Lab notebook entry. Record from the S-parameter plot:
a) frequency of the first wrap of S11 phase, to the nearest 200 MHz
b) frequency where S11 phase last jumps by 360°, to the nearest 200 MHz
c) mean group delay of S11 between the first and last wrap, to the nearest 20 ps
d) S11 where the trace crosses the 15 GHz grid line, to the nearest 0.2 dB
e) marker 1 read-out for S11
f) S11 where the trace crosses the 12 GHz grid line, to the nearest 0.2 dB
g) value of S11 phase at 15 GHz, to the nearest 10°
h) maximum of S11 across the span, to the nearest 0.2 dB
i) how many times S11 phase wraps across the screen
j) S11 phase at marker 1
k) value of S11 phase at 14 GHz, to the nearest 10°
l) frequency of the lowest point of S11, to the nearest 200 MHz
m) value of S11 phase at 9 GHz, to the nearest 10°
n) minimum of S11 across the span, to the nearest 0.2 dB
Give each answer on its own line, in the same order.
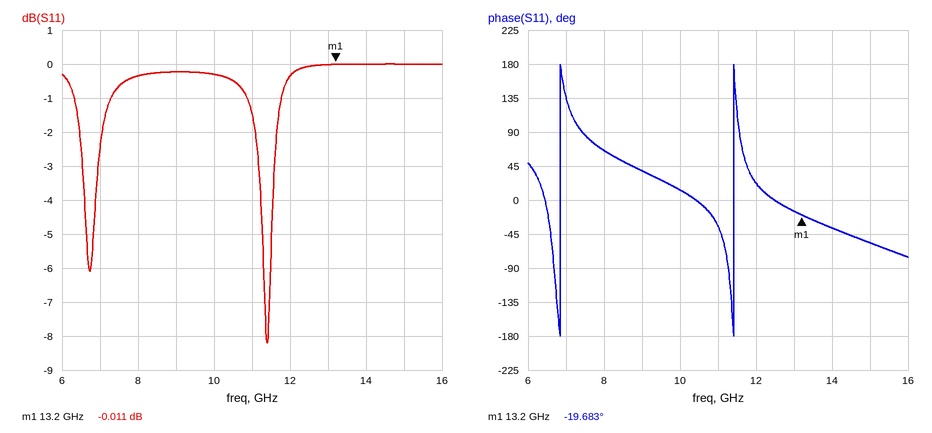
6.8 GHz
11.4 GHz
220 ps
0.0 dB
-0.011 dB
-0.4 dB
-60°
0.0 dB
2
-19.683°
-40°
11.4 GHz
40°
-8.2 dB
